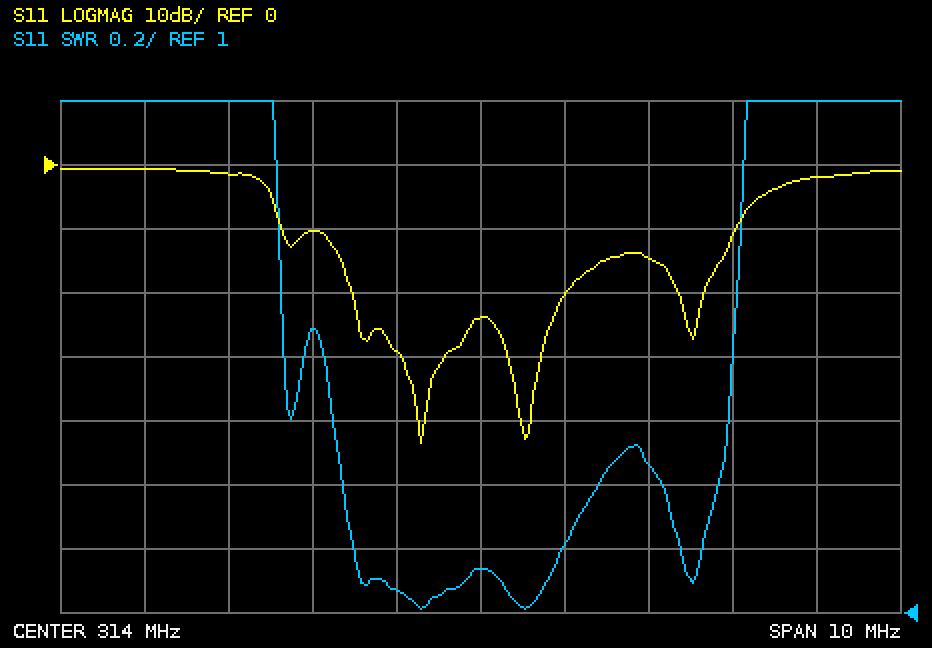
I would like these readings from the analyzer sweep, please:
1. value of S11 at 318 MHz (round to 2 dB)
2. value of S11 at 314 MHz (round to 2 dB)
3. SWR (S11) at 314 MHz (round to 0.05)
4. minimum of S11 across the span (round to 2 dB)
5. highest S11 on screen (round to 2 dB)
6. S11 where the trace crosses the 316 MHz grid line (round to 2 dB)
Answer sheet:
-2 dB
-24 dB
1.15
-44 dB
0 dB
-14 dB
